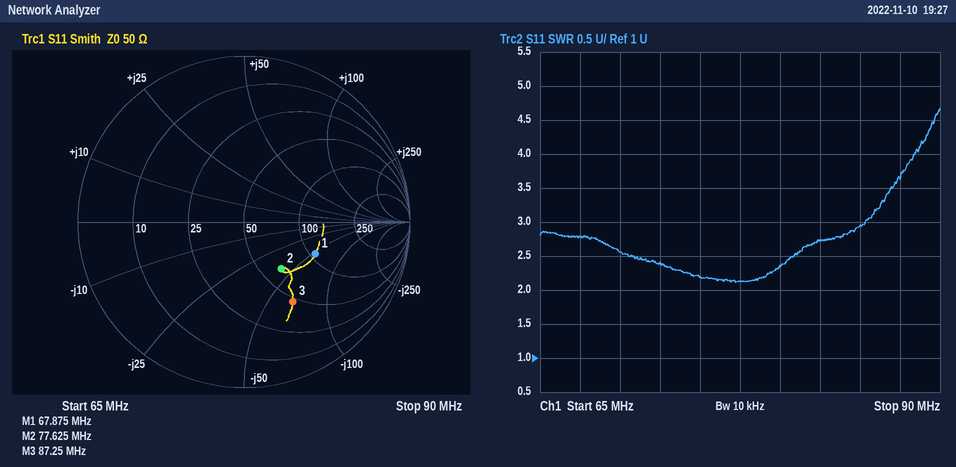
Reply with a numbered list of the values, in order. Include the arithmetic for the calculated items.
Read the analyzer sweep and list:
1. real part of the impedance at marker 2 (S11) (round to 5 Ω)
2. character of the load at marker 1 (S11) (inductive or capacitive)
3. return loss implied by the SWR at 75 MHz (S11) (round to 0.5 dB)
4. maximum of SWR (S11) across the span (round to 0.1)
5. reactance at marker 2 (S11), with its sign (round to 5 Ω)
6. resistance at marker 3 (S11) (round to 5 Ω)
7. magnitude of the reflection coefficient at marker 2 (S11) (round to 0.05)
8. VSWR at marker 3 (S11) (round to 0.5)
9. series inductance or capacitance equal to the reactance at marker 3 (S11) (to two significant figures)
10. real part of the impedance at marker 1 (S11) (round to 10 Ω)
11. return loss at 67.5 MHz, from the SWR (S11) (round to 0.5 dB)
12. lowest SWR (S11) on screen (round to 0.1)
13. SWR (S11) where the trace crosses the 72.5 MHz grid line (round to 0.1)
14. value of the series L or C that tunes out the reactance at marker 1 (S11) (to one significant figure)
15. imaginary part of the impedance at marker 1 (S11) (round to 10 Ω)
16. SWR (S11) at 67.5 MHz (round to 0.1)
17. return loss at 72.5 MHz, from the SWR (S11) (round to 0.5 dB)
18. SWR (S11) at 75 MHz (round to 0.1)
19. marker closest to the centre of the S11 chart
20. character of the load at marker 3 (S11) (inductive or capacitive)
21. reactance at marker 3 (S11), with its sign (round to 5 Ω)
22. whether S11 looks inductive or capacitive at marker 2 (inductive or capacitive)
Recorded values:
1. 65 Ω
2. capacitive
3. −20 log10((2.2 − 1)/(2.2 + 1)) ≈ 8.5 dB
4. 4.7
5. -40 Ω
6. 45 Ω
7. 0.35
8. 3.5
9. C = 1/(2π × 87.25 MHz × 65 Ω) ≈ 28 pF
10. 110 Ω
11. −20 log10((2.8 − 1)/(2.8 + 1)) ≈ 6.5 dB
12. 2.1
13. 2.4
14. L = 50 Ω/(2π × 67.875 MHz) ≈ 117 nH, so 100 nH to one significant figure
15. -50 Ω
16. 2.8
17. −20 log10((2.4 − 1)/(2.4 + 1)) ≈ 7.71 dB, so 7.5 dB to the nearest 0.5 dB
18. 2.2
19. marker 2
20. capacitive
21. -65 Ω
22. capacitive
